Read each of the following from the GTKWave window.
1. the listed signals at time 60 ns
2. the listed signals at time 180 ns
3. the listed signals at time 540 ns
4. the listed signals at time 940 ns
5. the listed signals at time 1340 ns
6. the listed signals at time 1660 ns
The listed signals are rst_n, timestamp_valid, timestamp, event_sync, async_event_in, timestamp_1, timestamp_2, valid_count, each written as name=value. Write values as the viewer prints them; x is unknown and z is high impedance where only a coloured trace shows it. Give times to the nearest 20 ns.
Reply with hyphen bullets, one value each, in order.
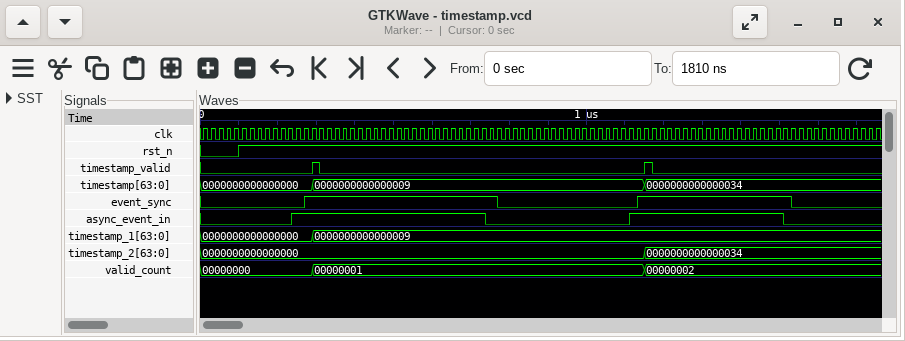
- rst_n=0, timestamp_valid=0, timestamp=0000000000000000, event_sync=0, async_event_in=0, timestamp_1=0000000000000000, timestamp_2=0000000000000000, valid_count=00000000
- rst_n=1, timestamp_valid=0, timestamp=0000000000000000, event_sync=0, async_event_in=0, timestamp_1=0000000000000000, timestamp_2=0000000000000000, valid_count=00000000
- rst_n=1, timestamp_valid=0, timestamp=0000000000000009, event_sync=1, async_event_in=1, timestamp_1=0000000000000009, timestamp_2=0000000000000000, valid_count=00000001
- rst_n=1, timestamp_valid=0, timestamp=0000000000000009, event_sync=0, async_event_in=0, timestamp_1=0000000000000009, timestamp_2=0000000000000000, valid_count=00000001
- rst_n=1, timestamp_valid=0, timestamp=0000000000000034, event_sync=1, async_event_in=1, timestamp_1=0000000000000009, timestamp_2=0000000000000034, valid_count=00000002
- rst_n=1, timestamp_valid=0, timestamp=0000000000000034, event_sync=0, async_event_in=0, timestamp_1=0000000000000009, timestamp_2=0000000000000034, valid_count=00000002
